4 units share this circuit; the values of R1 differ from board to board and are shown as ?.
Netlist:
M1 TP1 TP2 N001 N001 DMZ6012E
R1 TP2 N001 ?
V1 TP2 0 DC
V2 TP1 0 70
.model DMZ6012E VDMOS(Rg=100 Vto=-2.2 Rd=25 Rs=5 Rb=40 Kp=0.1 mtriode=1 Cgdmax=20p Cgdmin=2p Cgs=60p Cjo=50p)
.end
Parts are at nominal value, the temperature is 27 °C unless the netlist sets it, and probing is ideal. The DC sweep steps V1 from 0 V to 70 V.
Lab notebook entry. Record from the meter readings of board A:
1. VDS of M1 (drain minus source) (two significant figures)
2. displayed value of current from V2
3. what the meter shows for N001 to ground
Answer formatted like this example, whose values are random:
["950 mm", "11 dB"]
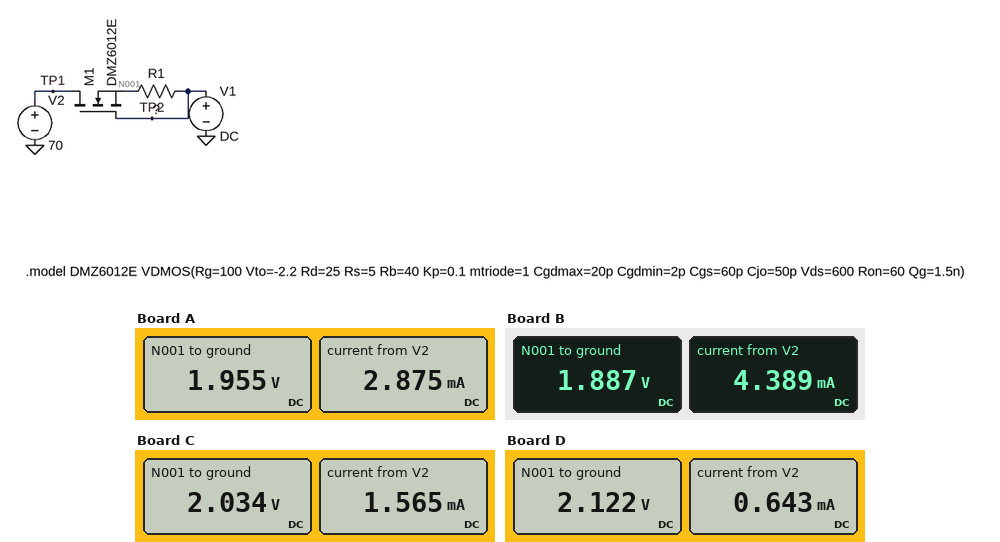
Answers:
["68 V", "2.875 mA", "1.955 V"]
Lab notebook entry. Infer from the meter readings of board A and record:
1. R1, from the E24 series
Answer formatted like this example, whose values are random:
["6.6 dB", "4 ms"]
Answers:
["680 Ω"]
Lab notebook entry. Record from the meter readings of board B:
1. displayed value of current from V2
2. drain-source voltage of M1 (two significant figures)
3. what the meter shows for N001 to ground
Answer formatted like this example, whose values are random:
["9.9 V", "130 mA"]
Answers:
["4.389 mA", "68 V", "1.887 V"]
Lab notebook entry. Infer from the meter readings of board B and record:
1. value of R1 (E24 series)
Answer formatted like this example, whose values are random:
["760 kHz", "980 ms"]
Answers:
["430 Ω"]
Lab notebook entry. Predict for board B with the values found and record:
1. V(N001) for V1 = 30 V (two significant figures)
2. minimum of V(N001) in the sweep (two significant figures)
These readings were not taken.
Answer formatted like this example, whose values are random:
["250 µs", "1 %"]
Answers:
["32 V", "1.9 V"]
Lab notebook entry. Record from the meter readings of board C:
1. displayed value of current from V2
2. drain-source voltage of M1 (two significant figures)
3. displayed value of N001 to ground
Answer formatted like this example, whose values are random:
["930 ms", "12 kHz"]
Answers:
["1.565 mA", "68 V", "2.034 V"]
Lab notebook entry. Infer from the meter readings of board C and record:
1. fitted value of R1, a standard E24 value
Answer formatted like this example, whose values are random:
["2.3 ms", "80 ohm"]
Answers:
["1.3 kΩ"]
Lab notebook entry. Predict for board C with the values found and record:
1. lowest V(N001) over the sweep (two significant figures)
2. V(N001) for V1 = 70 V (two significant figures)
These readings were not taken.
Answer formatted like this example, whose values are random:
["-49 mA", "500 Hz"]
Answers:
["2.0 V", "70 V"]
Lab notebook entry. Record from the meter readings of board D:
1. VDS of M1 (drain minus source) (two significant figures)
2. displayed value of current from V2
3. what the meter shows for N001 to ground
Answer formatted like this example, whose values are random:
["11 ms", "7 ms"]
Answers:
["68 V", "0.643 mA", "2.122 V"]
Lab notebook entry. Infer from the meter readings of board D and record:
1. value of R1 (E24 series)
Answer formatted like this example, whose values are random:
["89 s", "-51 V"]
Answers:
["3.3 kΩ"]
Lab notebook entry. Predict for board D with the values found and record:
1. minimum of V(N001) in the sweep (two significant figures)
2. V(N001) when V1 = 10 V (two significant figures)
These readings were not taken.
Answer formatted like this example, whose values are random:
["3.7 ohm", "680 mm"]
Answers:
["2.1 V", "12 V"]
